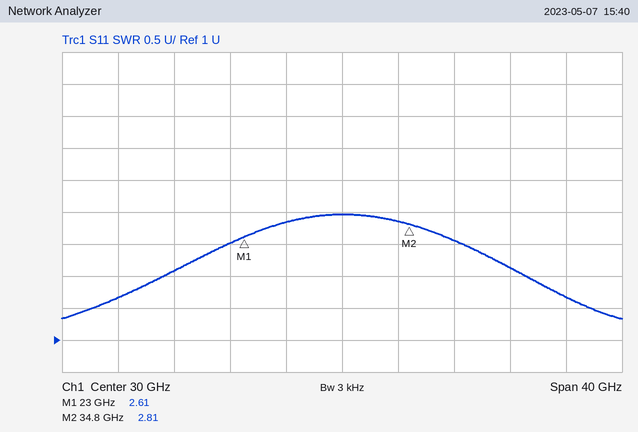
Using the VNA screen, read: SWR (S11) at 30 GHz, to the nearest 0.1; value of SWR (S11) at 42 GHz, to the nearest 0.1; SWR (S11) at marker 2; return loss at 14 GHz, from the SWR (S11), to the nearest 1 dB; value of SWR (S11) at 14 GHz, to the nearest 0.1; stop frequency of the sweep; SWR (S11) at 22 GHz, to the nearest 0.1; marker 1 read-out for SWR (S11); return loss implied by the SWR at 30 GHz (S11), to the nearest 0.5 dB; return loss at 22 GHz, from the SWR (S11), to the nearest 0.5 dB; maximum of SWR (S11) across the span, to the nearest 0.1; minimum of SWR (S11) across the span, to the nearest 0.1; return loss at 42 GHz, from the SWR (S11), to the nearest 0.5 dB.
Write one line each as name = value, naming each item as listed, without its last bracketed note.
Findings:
SWR (S11) at 30 GHz, to the nearest 0.1 = 3.0
value of SWR (S11) at 42 GHz, to the nearest 0.1 = 2.1
SWR (S11) at marker 2 = 2.81
return loss at 14 GHz, from the SWR (S11), to the nearest 1 dB = 12 dB
value of SWR (S11) at 14 GHz, to the nearest 0.1 = 1.7
stop frequency of the sweep = 50 GHz
SWR (S11) at 22 GHz, to the nearest 0.1 = 2.5
marker 1 read-out for SWR = 2.61
return loss implied by the SWR at 30 GHz (S11), to the nearest 0.5 dB = 6.0 dB
return loss at 22 GHz, from the SWR (S11), to the nearest 0.5 dB = 7.5 dB
maximum of SWR (S11) across the span, to the nearest 0.1 = 3.0
minimum of SWR (S11) across the span, to the nearest 0.1 = 1.3
return loss at 42 GHz, from the SWR (S11), to the nearest 0.5 dB = 9.0 dB
